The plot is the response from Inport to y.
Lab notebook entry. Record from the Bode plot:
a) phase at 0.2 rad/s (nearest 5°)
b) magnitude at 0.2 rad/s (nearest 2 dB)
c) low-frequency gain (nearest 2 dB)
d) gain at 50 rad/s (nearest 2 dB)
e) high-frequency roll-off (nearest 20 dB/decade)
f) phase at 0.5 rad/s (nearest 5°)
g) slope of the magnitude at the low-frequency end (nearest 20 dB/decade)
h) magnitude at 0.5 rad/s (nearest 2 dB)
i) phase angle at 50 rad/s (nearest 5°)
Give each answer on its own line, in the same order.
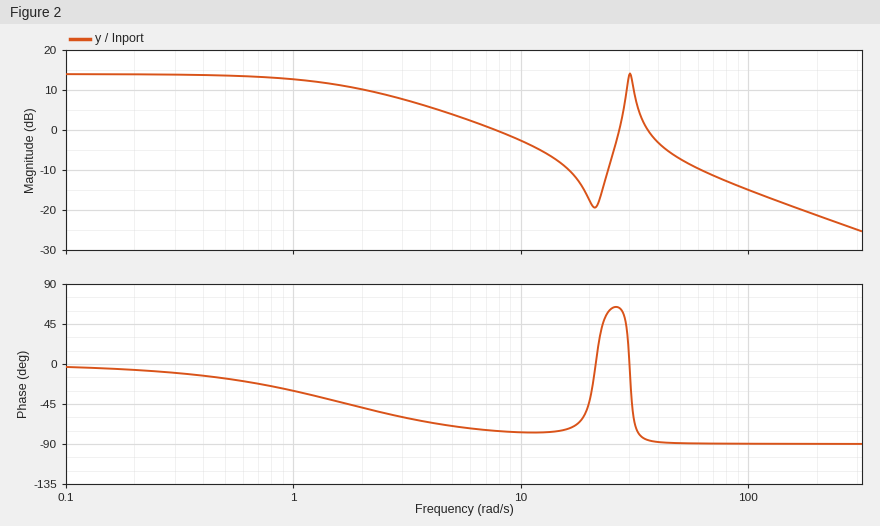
-5°
14 dB
14 dB
-8 dB
-20 dB/decade
-15°
0 dB/decade
14 dB
-90°
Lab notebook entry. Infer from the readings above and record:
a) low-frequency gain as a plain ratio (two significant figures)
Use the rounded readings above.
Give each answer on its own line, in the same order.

5.0
